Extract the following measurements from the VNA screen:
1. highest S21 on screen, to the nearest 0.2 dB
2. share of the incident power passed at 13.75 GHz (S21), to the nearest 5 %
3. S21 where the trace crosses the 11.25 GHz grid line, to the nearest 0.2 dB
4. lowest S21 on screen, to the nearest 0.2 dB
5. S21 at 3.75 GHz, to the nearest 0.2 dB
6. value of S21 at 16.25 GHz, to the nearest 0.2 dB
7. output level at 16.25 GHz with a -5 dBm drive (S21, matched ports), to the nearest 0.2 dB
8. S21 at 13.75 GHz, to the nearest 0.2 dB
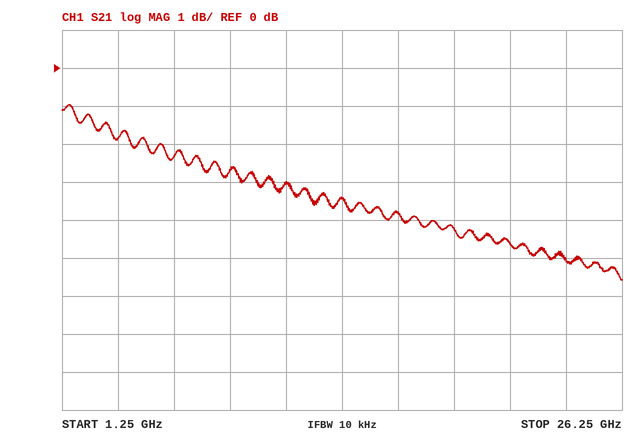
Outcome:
-1.0 dB
45 %
-3.0 dB
-5.6 dB
-1.8 dB
-3.8 dB
-8.8 dBm
-3.4 dB
